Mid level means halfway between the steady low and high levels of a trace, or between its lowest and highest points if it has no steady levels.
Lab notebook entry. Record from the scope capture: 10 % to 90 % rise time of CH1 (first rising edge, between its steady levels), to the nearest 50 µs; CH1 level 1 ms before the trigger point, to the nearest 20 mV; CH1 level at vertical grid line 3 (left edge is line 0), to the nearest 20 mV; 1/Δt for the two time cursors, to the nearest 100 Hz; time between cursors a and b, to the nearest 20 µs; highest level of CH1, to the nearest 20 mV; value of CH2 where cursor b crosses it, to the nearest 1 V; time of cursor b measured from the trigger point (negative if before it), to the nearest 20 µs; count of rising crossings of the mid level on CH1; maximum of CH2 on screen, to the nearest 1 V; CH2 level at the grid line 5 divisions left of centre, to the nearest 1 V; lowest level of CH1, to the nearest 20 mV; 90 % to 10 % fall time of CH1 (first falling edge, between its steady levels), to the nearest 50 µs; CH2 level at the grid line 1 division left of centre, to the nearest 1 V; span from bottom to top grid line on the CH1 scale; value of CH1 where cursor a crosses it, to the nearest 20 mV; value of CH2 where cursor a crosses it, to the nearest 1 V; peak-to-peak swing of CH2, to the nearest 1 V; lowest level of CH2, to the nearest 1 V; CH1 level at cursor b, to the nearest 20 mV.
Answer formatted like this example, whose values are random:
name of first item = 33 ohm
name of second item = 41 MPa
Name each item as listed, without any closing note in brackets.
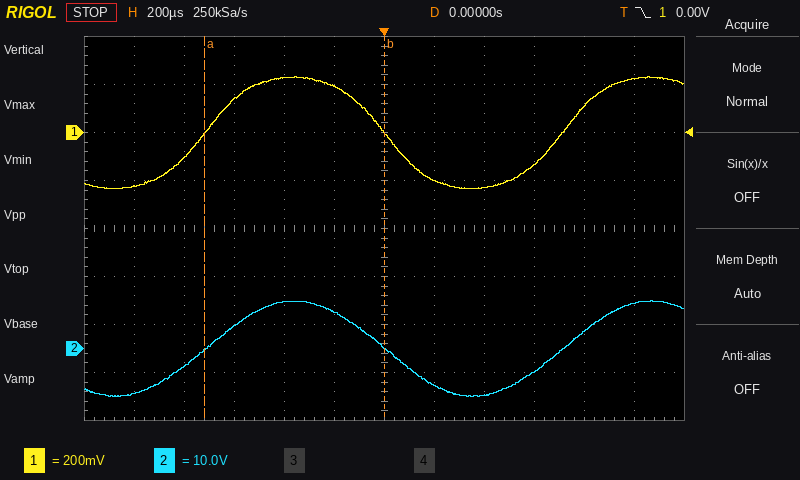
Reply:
10 % to 90 % rise time of CH1 (first rising edge, between its steady levels), to the nearest 50 µs = 350 µs
CH1 level 1 ms before the trigger point, to the nearest 20 mV = -220 mV
CH1 level at vertical grid line 3 (left edge is line 0), to the nearest 20 mV = 140 mV
1/Δt for the two time cursors, to the nearest 100 Hz = 1.4 kHz
time between cursors a and b, to the nearest 20 µs = 720 µs
highest level of CH1, to the nearest 20 mV = 240 mV
value of CH2 where cursor b crosses it, to the nearest 1 V = 0 V
time of cursor b measured from the trigger point (negative if before it), to the nearest 20 µs = 0 µs
count of rising crossings of the mid level on CH1 = 2
maximum of CH2 on screen, to the nearest 1 V = 10 V
CH2 level at the grid line 5 divisions left of centre, to the nearest 1 V = -9 V
lowest level of CH1, to the nearest 20 mV = -240 mV
90 % to 10 % fall time of CH1 (first falling edge, between its steady levels), to the nearest 50 µs = 350 µs
CH2 level at the grid line 1 division left of centre, to the nearest 1 V = 8 V
span from bottom to top grid line on the CH1 scale = 1.6 V
value of CH1 where cursor a crosses it, to the nearest 20 mV = 0 mV
value of CH2 where cursor a crosses it, to the nearest 1 V = 0 V
peak-to-peak swing of CH2, to the nearest 1 V = 20 V
lowest level of CH2, to the nearest 1 V = -10 V
CH1 level at cursor b, to the nearest 20 mV = 0 mV
